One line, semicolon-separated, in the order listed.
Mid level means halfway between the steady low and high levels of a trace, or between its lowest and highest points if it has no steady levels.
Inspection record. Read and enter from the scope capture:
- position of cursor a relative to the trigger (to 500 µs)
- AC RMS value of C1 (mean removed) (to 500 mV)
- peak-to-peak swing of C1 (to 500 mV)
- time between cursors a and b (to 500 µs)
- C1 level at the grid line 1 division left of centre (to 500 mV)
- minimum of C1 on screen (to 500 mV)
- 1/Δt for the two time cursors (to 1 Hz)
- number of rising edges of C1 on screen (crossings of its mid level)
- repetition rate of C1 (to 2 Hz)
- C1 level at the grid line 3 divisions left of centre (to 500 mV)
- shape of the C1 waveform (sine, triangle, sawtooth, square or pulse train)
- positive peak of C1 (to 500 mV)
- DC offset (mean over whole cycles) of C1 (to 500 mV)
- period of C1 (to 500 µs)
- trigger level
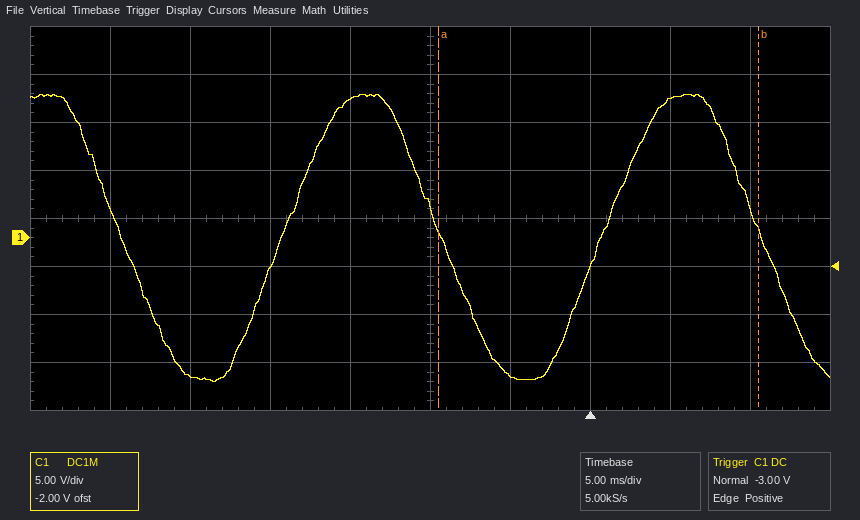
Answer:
-9.5 ms; 10.5 V; 30.0 V; 20.0 ms; 14.5 V; -15.0 V; 50 Hz; 2; 50 Hz; -14.5 V; sine; 15.0 V; 0.0 V; 20.0 ms; -3.00 V
